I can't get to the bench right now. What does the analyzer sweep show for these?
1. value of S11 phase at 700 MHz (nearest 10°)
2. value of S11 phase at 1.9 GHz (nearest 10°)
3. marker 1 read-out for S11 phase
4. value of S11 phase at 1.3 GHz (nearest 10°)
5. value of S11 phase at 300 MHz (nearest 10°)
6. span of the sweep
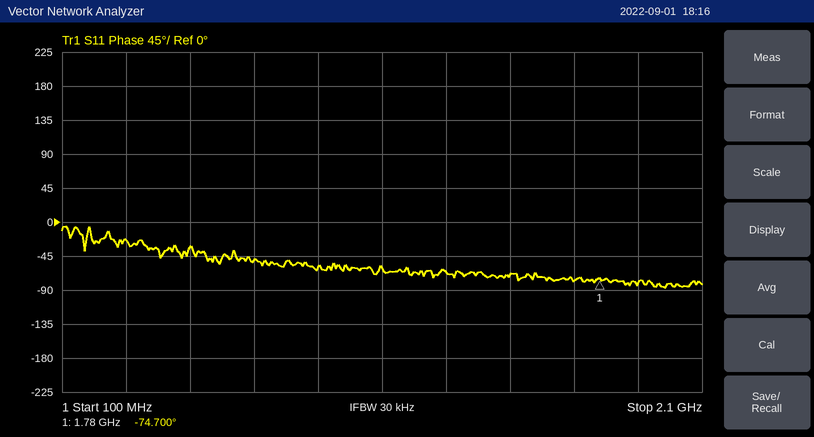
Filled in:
-50°
-80°
-74.700°
-70°
-20°
2 GHz
